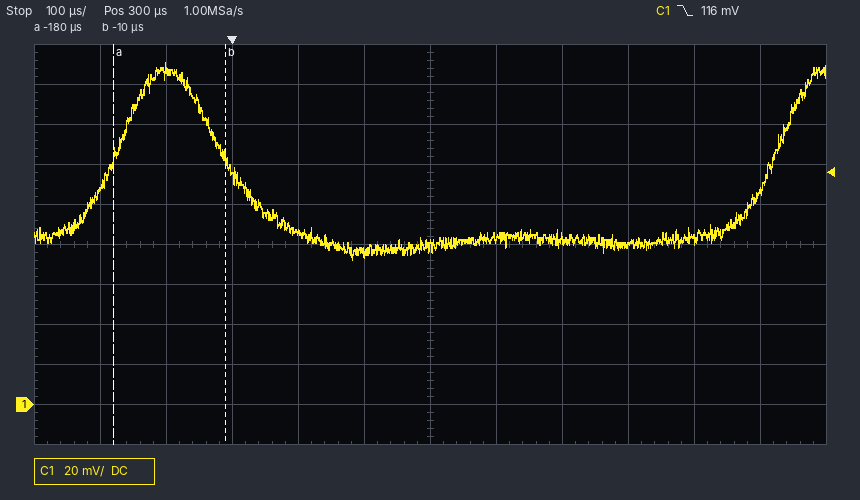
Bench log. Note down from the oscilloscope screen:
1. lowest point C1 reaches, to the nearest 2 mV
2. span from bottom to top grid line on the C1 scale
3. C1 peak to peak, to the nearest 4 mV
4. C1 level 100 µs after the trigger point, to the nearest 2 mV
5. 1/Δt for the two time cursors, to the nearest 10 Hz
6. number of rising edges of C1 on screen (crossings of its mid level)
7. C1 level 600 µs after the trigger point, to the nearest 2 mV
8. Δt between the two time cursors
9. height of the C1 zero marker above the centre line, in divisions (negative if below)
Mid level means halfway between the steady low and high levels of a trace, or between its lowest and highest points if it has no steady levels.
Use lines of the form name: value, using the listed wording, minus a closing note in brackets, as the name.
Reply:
lowest point C1 reaches, to the nearest 2 mV: 72 mV
span from bottom to top grid line on the C1 scale: 200 mV
C1 peak to peak, to the nearest 4 mV: 100 mV
C1 level 100 µs after the trigger point, to the nearest 2 mV: 86 mV
1/Δt for the two time cursors, to the nearest 10 Hz: 5.88 kHz
number of rising edges of C1 on screen: 2
C1 level 600 µs after the trigger point, to the nearest 2 mV: 80 mV
Δt between the two time cursors: 170 µs
height of the C1 zero marker above the centre line, in divisions: -4.0 div
